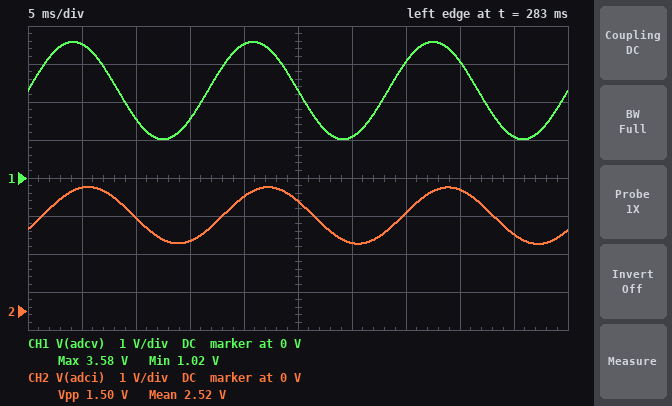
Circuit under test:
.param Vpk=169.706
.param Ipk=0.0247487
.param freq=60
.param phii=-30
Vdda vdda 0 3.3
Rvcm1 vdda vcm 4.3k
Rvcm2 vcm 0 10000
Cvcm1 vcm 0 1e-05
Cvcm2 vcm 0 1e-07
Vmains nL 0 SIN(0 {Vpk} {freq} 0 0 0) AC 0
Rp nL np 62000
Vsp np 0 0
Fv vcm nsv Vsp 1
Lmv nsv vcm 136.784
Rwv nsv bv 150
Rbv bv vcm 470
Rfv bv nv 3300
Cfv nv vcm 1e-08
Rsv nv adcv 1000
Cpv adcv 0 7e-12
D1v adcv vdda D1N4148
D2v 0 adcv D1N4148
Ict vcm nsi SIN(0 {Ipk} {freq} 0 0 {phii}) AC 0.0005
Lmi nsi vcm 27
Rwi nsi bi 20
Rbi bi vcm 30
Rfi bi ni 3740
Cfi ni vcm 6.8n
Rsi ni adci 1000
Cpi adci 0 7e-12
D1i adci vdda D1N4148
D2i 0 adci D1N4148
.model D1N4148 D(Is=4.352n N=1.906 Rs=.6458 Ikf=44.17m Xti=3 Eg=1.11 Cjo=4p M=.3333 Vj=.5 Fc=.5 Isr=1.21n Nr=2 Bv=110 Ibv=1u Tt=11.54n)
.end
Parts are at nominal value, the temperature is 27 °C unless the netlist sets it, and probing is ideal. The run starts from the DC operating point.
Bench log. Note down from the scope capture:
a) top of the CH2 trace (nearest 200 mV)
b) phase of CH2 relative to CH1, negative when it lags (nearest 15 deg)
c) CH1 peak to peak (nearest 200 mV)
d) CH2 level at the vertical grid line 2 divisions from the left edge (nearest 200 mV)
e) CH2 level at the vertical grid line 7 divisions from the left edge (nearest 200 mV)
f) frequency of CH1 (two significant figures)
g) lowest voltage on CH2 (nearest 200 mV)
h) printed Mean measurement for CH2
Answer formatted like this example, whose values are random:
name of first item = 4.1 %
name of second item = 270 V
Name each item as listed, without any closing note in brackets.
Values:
top of the CH2 trace = 3.2 V
phase of CH2 relative to CH1, negative when it lags = -30 deg
CH1 peak to peak = 2.6 V
CH2 level at the vertical grid line 2 divisions from the left edge = 2.4 V
CH2 level at the vertical grid line 7 divisions from the left edge = 2.6 V
frequency of CH1 = 60 Hz
lowest voltage on CH2 = 1.8 V
printed Mean measurement for CH2 = 2.52 V
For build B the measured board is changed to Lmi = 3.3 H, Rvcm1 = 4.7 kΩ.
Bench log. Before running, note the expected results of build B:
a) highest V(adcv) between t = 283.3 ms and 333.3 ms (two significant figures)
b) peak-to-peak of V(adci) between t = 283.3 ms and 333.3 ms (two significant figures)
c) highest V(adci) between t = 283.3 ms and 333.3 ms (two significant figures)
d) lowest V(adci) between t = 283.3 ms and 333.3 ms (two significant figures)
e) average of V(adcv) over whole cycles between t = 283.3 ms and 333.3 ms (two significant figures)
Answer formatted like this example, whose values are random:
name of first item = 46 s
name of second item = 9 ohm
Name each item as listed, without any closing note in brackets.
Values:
highest V(adcv) between t = 283.3 ms and 333.3 ms = 3.5 V
peak-to-peak of V(adci) between t = 283.3 ms and 333.3 ms = 1.5 V
highest V(adci) between t = 283.3 ms and 333.3 ms = 3.0 V
lowest V(adci) between t = 283.3 ms and 333.3 ms = 1.5 V
average of V(adcv) over whole cycles between t = 283.3 ms and 333.3 ms = 2.2 V
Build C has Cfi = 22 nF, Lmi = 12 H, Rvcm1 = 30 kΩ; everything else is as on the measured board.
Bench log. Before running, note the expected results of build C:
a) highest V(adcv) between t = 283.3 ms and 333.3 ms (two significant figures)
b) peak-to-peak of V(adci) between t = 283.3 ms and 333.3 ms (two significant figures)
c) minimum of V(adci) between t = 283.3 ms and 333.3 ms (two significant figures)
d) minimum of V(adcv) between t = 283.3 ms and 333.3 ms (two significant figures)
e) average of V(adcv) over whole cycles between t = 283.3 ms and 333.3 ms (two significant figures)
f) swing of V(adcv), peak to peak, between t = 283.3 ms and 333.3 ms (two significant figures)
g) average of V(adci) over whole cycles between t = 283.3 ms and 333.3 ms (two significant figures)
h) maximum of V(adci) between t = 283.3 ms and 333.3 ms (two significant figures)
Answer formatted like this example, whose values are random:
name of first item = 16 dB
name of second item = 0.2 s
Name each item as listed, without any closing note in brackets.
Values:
highest V(adcv) between t = 283.3 ms and 333.3 ms = 2.1 V
peak-to-peak of V(adci) between t = 283.3 ms and 333.3 ms = 1.5 V
minimum of V(adci) between t = 283.3 ms and 333.3 ms = 190 mV
minimum of V(adcv) between t = 283.3 ms and 333.3 ms = -390 mV
average of V(adcv) over whole cycles between t = 283.3 ms and 333.3 ms = 840 mV
swing of V(adcv), peak to peak, between t = 283.3 ms and 333.3 ms = 2.5 V
average of V(adci) over whole cycles between t = 283.3 ms and 333.3 ms = 940 mV
maximum of V(adci) between t = 283.3 ms and 333.3 ms = 1.7 V
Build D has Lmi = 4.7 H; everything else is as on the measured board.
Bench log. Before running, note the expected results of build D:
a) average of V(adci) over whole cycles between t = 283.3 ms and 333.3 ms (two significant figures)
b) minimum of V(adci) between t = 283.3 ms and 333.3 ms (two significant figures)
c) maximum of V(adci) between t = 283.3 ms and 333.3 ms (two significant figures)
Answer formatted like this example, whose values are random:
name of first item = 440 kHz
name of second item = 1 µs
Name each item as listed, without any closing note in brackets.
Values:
average of V(adci) over whole cycles between t = 283.3 ms and 333.3 ms = 2.3 V
minimum of V(adci) between t = 283.3 ms and 333.3 ms = 1.6 V
maximum of V(adci) between t = 283.3 ms and 333.3 ms = 3.1 V
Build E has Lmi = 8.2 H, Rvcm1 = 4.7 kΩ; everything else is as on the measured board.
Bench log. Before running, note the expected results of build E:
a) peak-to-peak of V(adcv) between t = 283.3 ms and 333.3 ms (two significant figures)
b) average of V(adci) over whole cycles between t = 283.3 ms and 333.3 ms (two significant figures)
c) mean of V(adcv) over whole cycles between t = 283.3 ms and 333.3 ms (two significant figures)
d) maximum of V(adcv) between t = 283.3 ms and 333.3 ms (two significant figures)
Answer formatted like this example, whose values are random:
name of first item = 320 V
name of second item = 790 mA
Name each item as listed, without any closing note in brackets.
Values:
peak-to-peak of V(adcv) between t = 283.3 ms and 333.3 ms = 2.6 V
average of V(adci) over whole cycles between t = 283.3 ms and 333.3 ms = 2.3 V
mean of V(adcv) over whole cycles between t = 283.3 ms and 333.3 ms = 2.2 V
maximum of V(adcv) between t = 283.3 ms and 333.3 ms = 3.5 V
